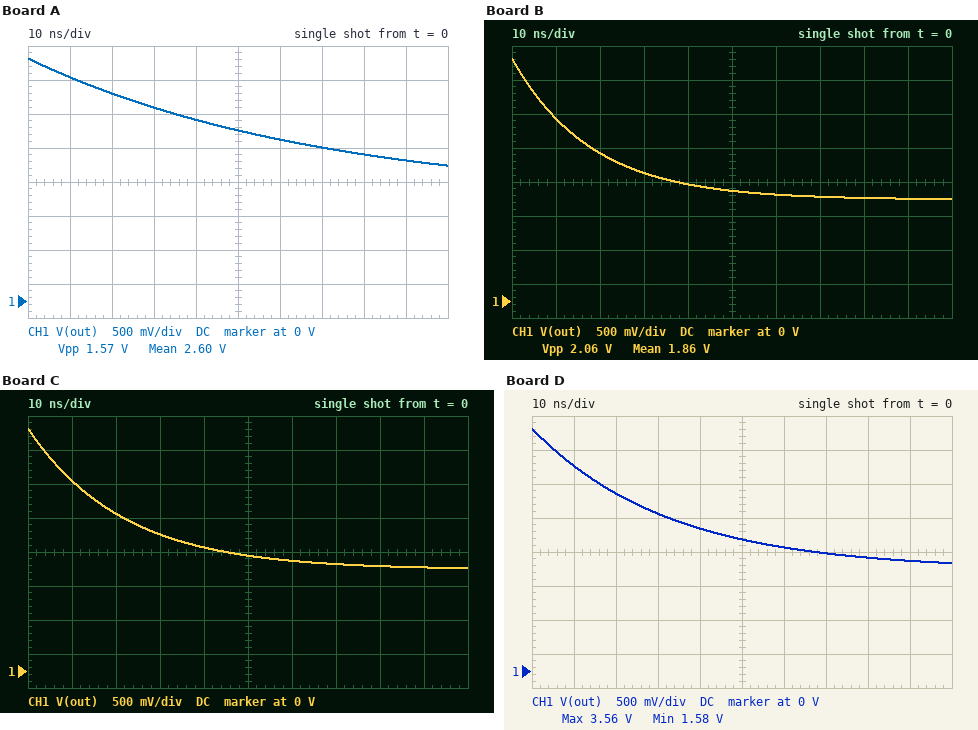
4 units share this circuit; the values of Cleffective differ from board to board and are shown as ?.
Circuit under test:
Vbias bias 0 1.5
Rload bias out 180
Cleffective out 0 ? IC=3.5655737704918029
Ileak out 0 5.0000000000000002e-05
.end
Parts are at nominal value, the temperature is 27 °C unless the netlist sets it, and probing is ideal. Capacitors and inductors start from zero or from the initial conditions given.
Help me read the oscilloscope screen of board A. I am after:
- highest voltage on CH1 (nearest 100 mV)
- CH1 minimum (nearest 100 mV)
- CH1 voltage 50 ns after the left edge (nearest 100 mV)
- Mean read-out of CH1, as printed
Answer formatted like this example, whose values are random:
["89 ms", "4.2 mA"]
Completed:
["3.6 V", "2.0 V", "2.5 V", "2.60 V"]
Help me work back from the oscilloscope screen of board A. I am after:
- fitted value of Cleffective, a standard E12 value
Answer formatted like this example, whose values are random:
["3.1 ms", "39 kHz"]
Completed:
["390 pF"]
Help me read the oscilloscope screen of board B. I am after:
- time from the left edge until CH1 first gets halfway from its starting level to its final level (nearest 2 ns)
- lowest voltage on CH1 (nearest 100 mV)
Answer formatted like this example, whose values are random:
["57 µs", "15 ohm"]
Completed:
["12 ns", "1.5 V"]
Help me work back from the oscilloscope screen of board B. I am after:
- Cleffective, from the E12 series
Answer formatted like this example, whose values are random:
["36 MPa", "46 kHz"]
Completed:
["100 pF"]
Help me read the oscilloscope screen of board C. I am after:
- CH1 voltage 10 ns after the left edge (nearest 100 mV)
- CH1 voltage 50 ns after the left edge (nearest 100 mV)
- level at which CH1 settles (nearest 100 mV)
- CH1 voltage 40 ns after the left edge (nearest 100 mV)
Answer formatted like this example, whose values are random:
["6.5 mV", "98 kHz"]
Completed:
["2.8 V", "1.7 V", "1.5 V", "1.8 V"]
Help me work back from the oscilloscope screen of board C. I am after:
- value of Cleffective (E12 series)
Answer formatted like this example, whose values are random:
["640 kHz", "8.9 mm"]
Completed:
["120 pF"]
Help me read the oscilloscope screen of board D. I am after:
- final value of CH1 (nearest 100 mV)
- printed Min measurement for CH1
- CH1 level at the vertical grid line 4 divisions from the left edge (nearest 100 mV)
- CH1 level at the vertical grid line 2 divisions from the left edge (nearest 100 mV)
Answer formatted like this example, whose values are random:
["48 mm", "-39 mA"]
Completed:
["1.6 V", "1.58 V", "2.1 V", "2.6 V"]
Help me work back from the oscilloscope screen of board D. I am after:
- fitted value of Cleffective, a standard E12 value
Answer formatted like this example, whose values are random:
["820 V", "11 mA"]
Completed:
["180 pF"]
